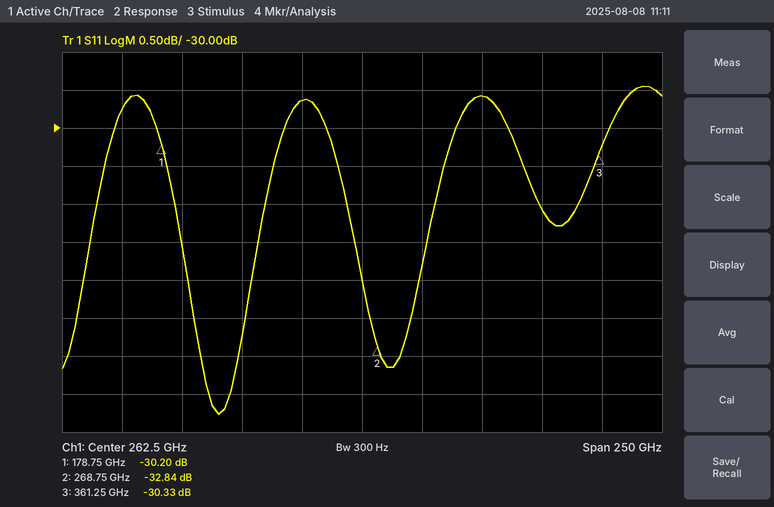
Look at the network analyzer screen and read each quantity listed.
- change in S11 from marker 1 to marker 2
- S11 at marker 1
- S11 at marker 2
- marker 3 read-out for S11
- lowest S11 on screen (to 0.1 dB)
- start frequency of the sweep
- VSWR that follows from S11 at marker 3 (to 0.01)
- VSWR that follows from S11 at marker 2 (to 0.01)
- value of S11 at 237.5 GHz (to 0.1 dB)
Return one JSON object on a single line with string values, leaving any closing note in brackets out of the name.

{"change in S11 from marker 1 to marker 2": "-2.64 dB", "S11 at marker 1": "-30.20 dB", "S11 at marker 2": "-32.84 dB", "marker 3 read-out for S11": "-30.33 dB", "lowest S11 on screen": "-33.8 dB", "start frequency of the sweep": "137.5 GHz", "VSWR that follows from S11 at marker 3": "1.06", "VSWR that follows from S11 at marker 2": "1.05", "value of S11 at 237.5 GHz": "-29.6 dB"}
